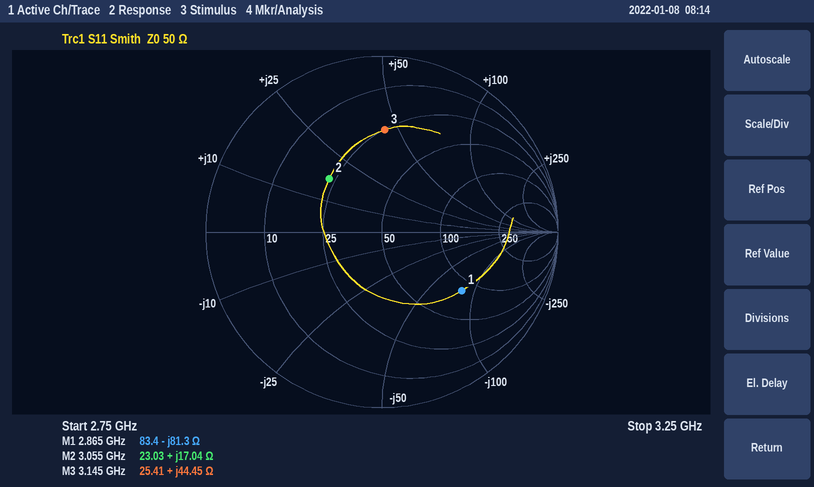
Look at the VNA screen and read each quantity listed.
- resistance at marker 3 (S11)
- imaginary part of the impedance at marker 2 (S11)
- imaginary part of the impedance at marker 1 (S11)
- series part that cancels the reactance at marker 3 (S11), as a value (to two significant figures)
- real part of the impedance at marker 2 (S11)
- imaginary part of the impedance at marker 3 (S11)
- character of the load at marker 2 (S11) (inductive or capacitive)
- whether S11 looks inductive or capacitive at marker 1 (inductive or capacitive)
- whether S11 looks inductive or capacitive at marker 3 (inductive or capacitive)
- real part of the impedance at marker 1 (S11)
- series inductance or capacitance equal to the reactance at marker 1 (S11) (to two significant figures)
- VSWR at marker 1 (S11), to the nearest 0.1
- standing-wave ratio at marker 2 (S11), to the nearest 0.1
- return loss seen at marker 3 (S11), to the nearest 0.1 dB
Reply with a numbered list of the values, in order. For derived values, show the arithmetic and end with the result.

1. 25.41 Ω
2. +17.04 Ω
3. -81.3 Ω
4. C = 1/(2π × 3.145 GHz × 44.45 Ω) ≈ 1.1 pF
5. 23.03 Ω
6. +44.45 Ω
7. inductive
8. capacitive
9. inductive
10. 83.4 Ω
11. C = 1/(2π × 2.865 GHz × 81.3 Ω) ≈ 683 fF, so 680 fF to two significant figures
12. 3.6
13. 2.5
14. 4.7 dB
